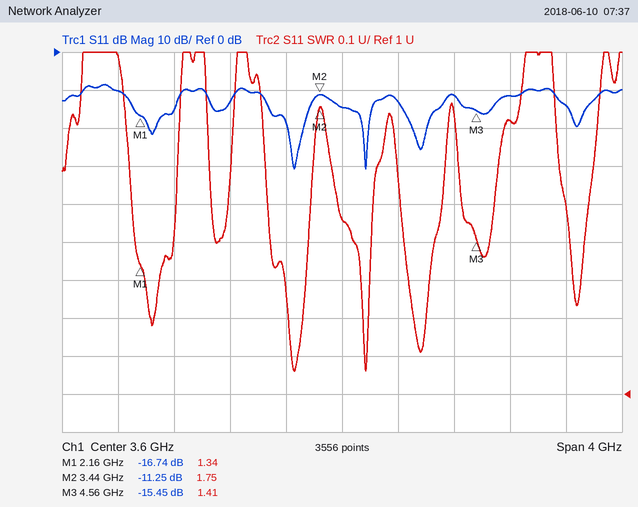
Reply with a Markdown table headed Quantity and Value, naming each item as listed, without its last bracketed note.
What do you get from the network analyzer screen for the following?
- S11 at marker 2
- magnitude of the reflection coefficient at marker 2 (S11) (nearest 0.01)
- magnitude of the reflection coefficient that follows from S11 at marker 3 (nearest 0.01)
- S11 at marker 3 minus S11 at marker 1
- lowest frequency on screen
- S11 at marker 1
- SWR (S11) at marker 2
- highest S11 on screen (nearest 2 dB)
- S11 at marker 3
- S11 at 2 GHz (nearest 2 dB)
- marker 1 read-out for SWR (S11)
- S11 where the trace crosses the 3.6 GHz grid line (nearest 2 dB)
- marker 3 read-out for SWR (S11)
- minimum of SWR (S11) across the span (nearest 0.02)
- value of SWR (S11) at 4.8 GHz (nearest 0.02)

| Quantity | Value |
|---|---|
| S11 at marker 2 | -11.25 dB |
| magnitude of the reflection coefficient at marker 2 (S11) | 0.27 |
| magnitude of the reflection coefficient that follows from S11 at marker 3 | 0.17 |
| S11 at marker 3 minus S11 at marker 1 | 1.29 dB |
| lowest frequency on screen | 1.6 GHz |
| S11 at marker 1 | -16.74 dB |
| SWR (S11) at marker 2 | 1.75 |
| highest S11 on screen | -8 dB |
| S11 at marker 3 | -15.45 dB |
| S11 at 2 GHz | -10 dB |
| marker 1 read-out for SWR | 1.34 |
| S11 where the trace crosses the 3.6 GHz grid line | -14 dB |
| marker 3 read-out for SWR | 1.41 |
| minimum of SWR (S11) across the span | 1.06 |
| value of SWR (S11) at 4.8 GHz | 1.72 |
